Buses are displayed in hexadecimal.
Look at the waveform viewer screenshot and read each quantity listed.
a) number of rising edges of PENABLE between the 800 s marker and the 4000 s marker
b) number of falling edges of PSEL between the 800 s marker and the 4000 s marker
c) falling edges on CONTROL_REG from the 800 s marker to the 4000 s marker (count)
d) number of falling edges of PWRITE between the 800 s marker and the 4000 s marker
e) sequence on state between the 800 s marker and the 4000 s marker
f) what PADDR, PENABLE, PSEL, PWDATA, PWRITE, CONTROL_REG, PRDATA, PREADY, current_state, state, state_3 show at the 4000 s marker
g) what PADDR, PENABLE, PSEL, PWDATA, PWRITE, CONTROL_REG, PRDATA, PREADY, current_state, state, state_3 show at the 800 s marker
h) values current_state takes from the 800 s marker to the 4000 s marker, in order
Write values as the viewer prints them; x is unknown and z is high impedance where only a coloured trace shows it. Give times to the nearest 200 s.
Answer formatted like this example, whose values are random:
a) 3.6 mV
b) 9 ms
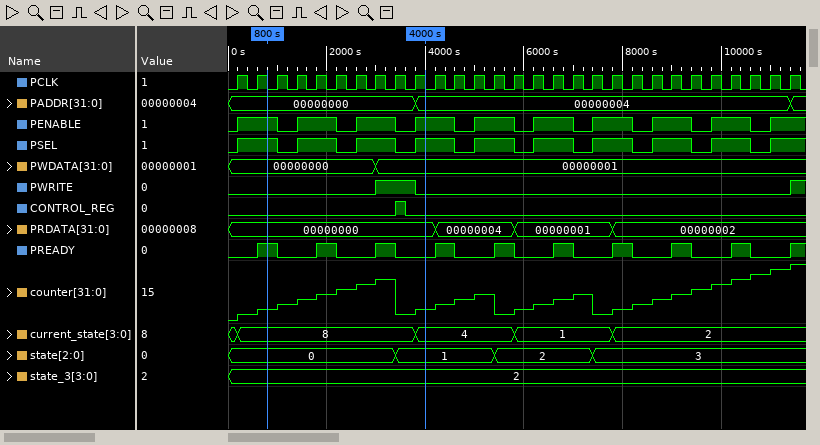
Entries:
a) 3
b) 3
c) 1
d) 1
e) 0, 1
f) PADDR=00000004, PENABLE=1, PSEL=1, PWDATA=00000001, PWRITE=0, CONTROL_REG=0, PRDATA=00000000, PREADY=0, current_state=4, state=1, state_3=2
g) PADDR=00000000, PENABLE=1, PSEL=1, PWDATA=00000000, PWRITE=0, CONTROL_REG=0, PRDATA=00000000, PREADY=1, current_state=8, state=0, state_3=2
h) 8, 4
